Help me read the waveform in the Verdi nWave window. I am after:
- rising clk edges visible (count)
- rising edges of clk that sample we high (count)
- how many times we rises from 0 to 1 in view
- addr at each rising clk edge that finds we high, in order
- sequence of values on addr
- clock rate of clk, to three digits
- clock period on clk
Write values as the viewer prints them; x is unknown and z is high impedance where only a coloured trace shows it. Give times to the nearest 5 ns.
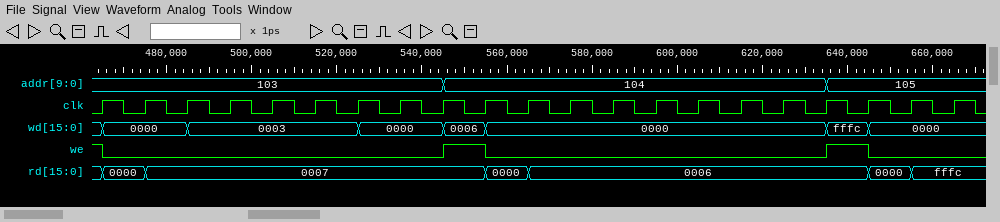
21
3
2
103, 104, 105
103, 104, 105
100 MHz
10 ns
